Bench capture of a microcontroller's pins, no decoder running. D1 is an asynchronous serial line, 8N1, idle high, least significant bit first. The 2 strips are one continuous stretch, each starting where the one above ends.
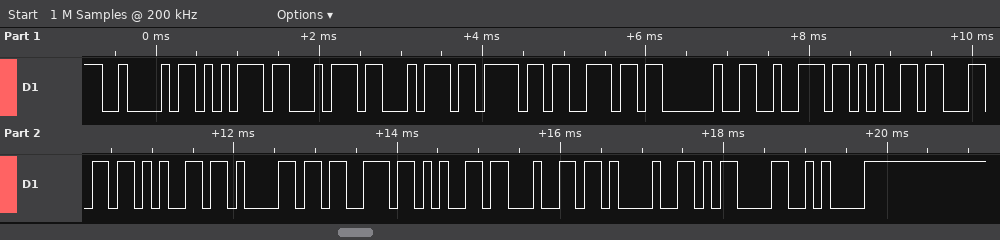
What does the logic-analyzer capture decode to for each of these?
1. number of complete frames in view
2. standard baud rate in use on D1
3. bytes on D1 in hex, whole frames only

18
9600 baud
0x42 0x75 0x74 0x74 0x6F 0x6E 0x20 0x72 0x65 0x6C 0x65 0x61 0x73 0x65 0x64 0x21 0x0D 0x0A
